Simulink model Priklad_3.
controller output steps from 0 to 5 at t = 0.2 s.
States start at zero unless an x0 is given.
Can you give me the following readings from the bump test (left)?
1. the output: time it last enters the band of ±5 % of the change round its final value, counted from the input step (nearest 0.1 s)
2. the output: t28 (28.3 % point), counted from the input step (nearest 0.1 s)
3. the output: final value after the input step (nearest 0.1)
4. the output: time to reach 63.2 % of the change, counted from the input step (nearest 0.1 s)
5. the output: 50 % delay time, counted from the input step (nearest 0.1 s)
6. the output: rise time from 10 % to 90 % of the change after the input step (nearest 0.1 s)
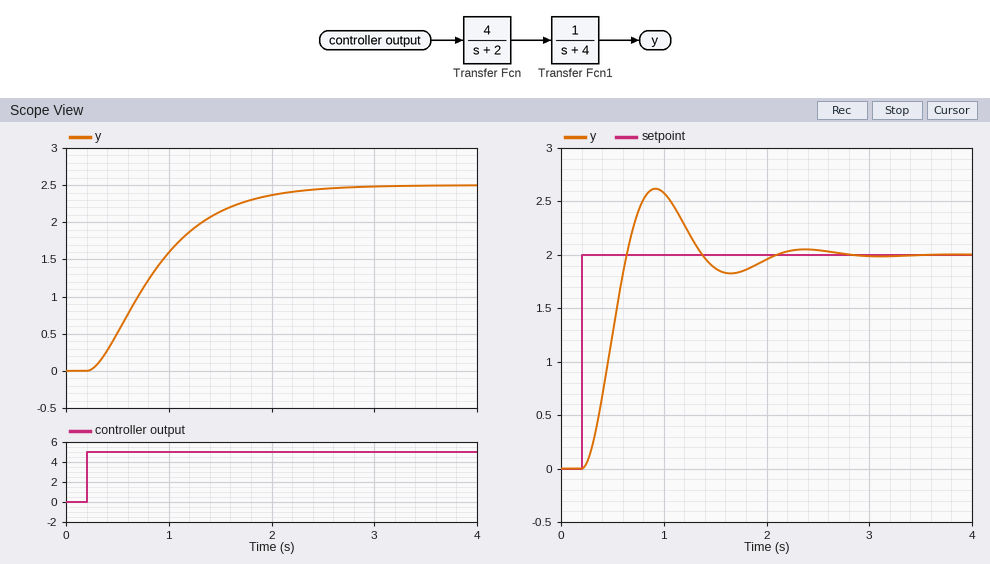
1.8 s
0.4 s
2.5
0.8 s
0.6 s
1.3 s
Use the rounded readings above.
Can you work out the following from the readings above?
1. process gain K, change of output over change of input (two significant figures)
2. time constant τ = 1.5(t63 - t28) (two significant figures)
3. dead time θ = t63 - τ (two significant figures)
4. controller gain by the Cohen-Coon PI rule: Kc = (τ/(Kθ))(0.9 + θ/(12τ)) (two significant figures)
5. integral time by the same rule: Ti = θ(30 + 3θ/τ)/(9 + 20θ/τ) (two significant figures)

0.50
0.60 s
0.20 s
5.6
0.40 s
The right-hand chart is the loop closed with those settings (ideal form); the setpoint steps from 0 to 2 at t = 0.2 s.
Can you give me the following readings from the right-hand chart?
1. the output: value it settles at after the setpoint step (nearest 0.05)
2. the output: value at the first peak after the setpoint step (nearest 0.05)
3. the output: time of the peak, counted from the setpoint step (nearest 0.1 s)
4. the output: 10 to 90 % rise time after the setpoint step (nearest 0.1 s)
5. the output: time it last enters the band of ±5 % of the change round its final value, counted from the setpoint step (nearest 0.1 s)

2.00
2.60
0.7 s
0.3 s
1.7 s
